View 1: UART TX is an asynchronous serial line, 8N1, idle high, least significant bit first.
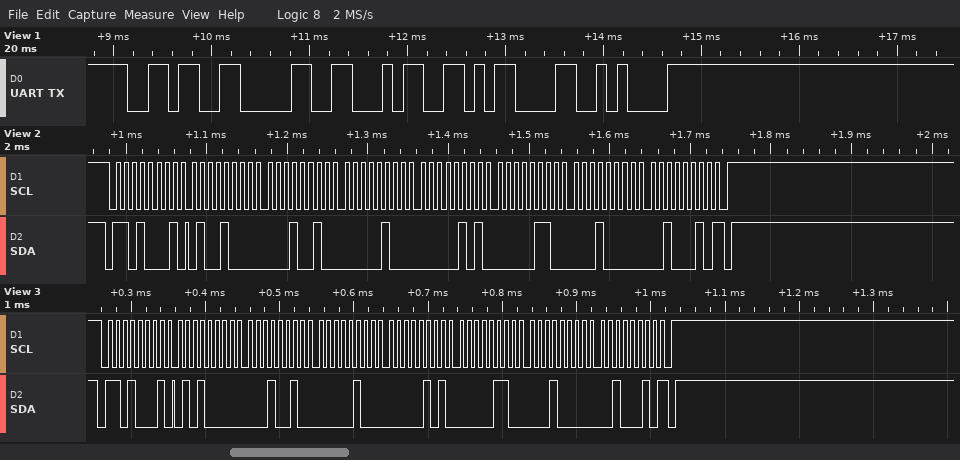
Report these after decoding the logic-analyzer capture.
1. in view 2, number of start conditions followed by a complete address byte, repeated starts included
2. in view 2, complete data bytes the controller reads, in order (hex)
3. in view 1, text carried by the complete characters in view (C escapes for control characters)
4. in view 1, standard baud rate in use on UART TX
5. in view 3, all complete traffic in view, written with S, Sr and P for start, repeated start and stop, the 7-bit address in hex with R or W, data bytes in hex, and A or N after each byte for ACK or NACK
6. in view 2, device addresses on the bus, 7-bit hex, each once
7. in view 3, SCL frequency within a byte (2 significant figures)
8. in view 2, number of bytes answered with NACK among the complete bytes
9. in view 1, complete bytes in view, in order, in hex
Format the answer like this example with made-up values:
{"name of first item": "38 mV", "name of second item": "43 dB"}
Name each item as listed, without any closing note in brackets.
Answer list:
{"in view 2, number of start conditions followed by a complete address byte, repeated starts included": "1", "in view 2, complete data bytes the controller reads, in order": "48 12 04 05 06 10 22", "in view 1, text carried by the complete characters in view": "\"604\\r\\n\"", "in view 1, standard baud rate in use on UART TX": "9600 baud", "in view 3, all complete traffic in view, written with S, Sr and P for start, repeated start and stop, the 7-bit address in hex with R or W, data bytes in hex, and A or N after each byte for ACK or NACK": "S 68R A 50 A 12 A 04 A 05 A 06 A 10 A 22 N P", "in view 2, device addresses on the bus, 7-bit hex, each once": "0x68", "in view 3, SCL frequency within a byte": "100 kHz", "in view 2, number of bytes answered with NACK among the complete bytes": "1", "in view 1, complete bytes in view, in order, in hex": "36 30 34 0D 0A"}
